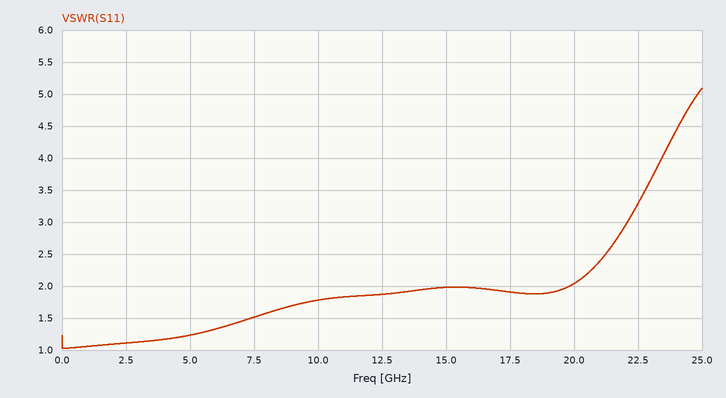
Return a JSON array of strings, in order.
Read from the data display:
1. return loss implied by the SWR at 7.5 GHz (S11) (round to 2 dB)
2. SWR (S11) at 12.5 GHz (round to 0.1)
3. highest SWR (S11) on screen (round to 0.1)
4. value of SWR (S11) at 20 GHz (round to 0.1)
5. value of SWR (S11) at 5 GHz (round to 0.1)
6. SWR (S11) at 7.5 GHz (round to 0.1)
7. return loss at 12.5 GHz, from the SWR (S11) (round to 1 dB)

["14 dB", "1.9", "5.1", "2.0", "1.2", "1.5", "10 dB"]
